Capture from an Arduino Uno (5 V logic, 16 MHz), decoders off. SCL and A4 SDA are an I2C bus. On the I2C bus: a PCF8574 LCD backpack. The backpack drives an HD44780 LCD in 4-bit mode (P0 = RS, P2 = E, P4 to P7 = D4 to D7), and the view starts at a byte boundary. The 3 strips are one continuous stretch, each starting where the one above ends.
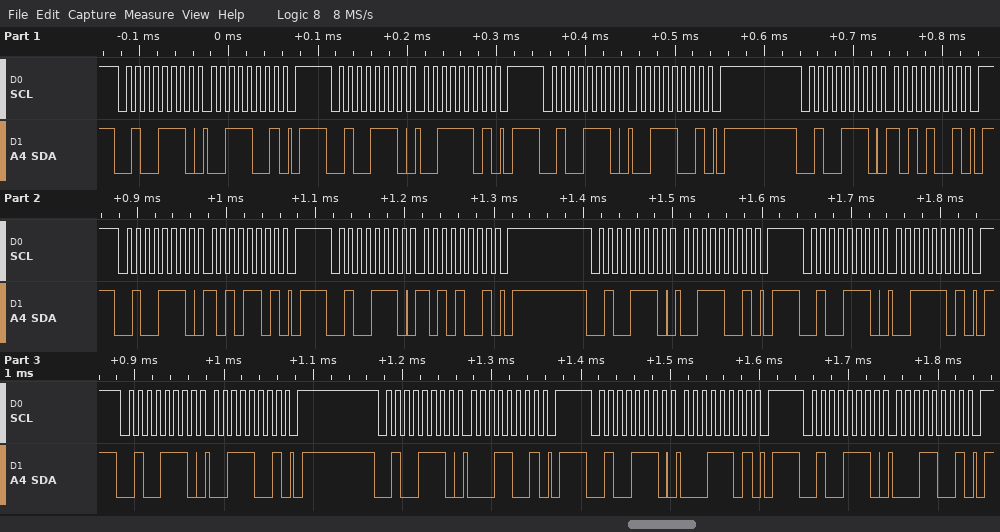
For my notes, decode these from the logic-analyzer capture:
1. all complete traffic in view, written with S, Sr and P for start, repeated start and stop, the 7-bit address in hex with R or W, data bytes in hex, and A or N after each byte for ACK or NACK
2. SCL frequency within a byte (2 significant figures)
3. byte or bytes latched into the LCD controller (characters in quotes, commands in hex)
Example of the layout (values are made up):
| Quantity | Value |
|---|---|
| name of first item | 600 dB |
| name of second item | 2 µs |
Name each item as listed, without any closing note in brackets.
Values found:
| Quantity | Value |
|---|---|
| all complete traffic in view, written with S, Sr and P for start, repeated start and stop, the 7-bit address in hex with R or W, data bytes in hex, and A or N after each byte for ACK or NACK | S 27W A 39 A P S 27W A 3D A P S 27W A 39 A P S 27W A A9 A P S 27W A AD A P S 27W A A9 A P S 27W A 39 A P S 27W A 3D A P S 27W A 39 A P S 27W A 19 A P S 27W A 1D A P S 27W A 19 A P |
| SCL frequency within a byte | 100 kHz |
| byte or bytes latched into the LCD controller | ':' '1' |
